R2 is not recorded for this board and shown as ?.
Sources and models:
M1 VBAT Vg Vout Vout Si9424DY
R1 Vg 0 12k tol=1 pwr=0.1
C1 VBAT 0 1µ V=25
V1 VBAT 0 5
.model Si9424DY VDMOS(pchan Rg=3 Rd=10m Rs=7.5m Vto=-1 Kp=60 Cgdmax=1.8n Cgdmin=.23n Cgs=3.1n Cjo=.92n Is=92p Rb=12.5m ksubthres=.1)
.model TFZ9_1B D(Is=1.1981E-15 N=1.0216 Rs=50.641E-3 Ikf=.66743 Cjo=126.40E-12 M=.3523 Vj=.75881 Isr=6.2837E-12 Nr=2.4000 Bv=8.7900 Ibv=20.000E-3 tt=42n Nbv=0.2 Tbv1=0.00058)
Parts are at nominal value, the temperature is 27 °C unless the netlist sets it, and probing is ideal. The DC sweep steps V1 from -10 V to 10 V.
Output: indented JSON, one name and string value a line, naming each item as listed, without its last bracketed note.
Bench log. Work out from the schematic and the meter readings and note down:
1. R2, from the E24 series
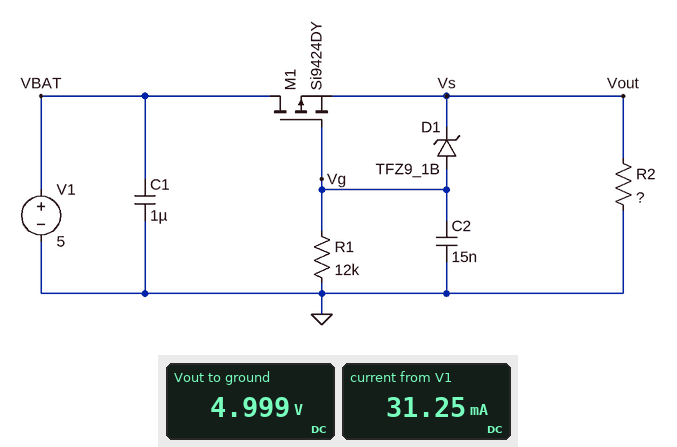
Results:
{
  "R2, from the E24 series": "160 Ω"
}
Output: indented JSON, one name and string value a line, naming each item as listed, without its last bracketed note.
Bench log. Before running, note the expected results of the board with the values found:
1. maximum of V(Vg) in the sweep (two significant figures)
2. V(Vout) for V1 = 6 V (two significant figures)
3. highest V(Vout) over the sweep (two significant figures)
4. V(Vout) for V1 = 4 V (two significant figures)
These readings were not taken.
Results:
{
  "maximum of V(Vg) in the sweep": "1.2 V",
  "V(Vout) for V1 = 6 V": "6.0 V",
  "highest V(Vout) over the sweep": "10 V",
  "V(Vout) for V1 = 4 V": "4.0 V"
}
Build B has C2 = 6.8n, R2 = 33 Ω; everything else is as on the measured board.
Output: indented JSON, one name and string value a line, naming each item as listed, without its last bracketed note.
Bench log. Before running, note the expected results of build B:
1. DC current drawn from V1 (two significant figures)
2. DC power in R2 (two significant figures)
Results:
{
  "DC current drawn from V1": "150 mA",
  "DC power in R2": "760 mW"
}
